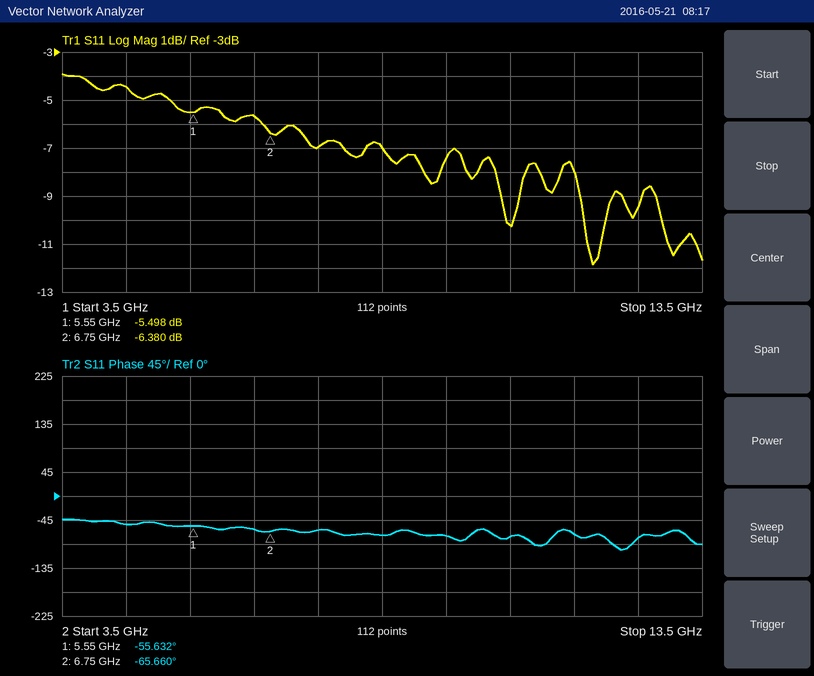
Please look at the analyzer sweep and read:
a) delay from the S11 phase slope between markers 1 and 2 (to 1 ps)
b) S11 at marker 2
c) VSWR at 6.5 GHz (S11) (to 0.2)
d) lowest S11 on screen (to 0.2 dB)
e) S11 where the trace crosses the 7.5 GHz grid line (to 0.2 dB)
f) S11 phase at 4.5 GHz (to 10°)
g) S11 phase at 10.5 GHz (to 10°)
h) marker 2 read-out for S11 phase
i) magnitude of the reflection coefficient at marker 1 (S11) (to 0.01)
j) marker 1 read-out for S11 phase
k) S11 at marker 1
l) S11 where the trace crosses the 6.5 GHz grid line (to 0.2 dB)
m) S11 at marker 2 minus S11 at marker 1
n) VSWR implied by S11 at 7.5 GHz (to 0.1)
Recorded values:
23 ps
-6.380 dB
3.2
-11.8 dB
-7.0 dB
-50°
-80°
-65.660°
0.53
-55.632°
-5.498 dB
-5.6 dB
-0.882 dB
2.6
